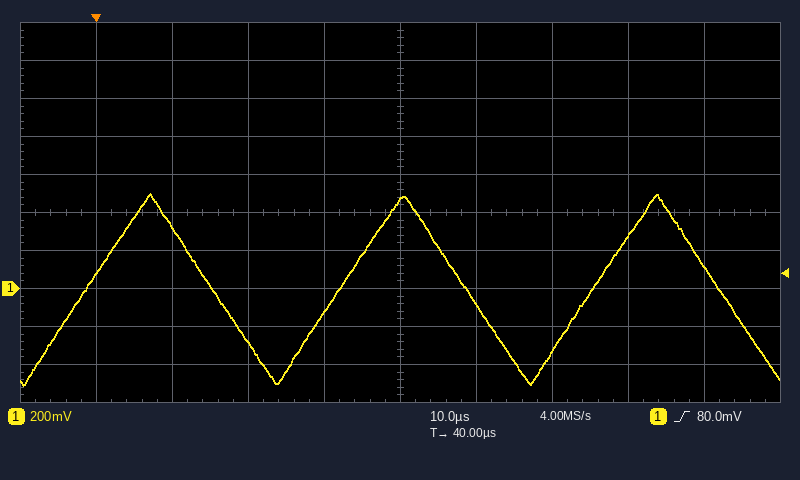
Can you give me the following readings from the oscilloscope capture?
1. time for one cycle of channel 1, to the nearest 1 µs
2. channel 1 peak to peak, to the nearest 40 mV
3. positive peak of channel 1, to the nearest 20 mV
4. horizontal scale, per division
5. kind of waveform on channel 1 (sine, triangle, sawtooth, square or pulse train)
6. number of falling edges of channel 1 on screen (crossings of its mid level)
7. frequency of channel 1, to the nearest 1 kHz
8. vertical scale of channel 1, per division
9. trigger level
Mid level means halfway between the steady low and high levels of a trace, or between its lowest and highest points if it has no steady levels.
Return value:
33 µs
1.00 V
500 mV
10 µs
triangle
3
30 kHz
200 mV
80.0 mV
